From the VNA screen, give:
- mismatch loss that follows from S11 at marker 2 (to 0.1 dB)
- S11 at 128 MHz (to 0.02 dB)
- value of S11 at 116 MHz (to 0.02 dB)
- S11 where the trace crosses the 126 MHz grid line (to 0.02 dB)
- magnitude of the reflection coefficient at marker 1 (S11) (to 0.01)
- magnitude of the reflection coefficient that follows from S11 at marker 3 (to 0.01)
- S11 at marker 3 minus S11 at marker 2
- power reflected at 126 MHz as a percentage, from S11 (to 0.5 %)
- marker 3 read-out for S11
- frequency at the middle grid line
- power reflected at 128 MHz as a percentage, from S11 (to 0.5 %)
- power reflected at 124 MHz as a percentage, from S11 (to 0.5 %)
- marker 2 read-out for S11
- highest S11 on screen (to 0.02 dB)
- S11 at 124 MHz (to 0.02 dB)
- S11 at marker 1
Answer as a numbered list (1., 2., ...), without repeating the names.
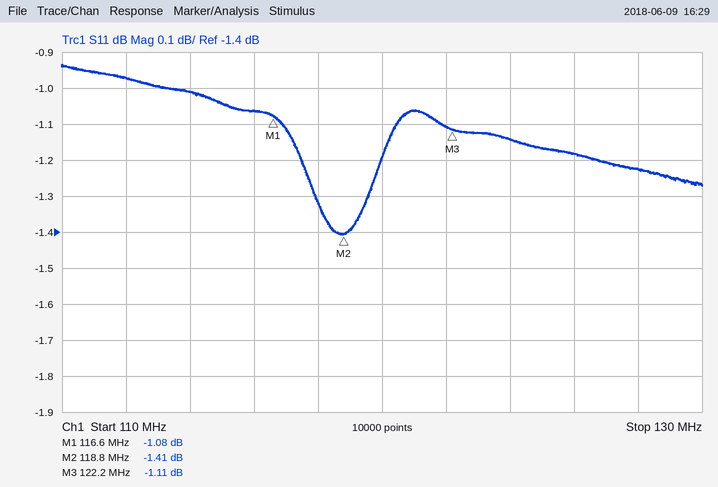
1. 5.6 dB
2. -1.22 dB
3. -1.06 dB
4. -1.18 dB
5. 0.88
6. 0.88
7. 0.30 dB
8. 76.0 %
9. -1.11 dB
10. 120 MHz
11. 75.5 %
12. 77.0 %
13. -1.41 dB
14. -0.94 dB
15. -1.14 dB
16. -1.08 dB
